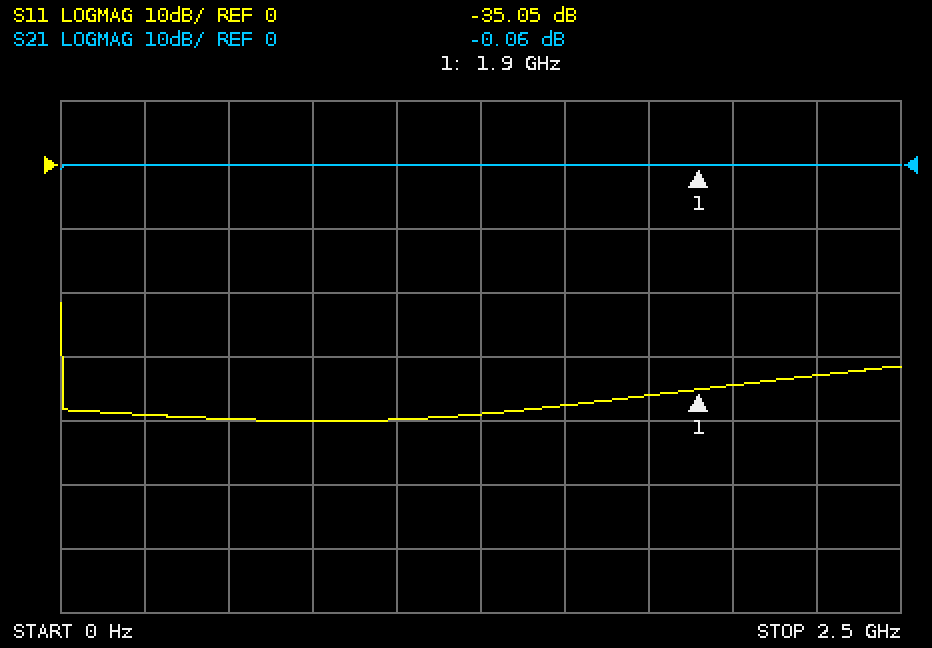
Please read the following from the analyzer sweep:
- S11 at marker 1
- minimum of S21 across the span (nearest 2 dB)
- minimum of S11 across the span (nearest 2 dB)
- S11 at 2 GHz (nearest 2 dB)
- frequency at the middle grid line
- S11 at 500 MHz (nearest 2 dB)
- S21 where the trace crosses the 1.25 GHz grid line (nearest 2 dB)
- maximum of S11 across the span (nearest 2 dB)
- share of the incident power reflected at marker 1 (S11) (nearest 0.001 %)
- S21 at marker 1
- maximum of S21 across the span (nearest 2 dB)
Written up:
-35.05 dB
0 dB
-40 dB
-34 dB
1.25 GHz
-40 dB
0 dB
-22 dB
0.031 %
-0.06 dB
0 dB
